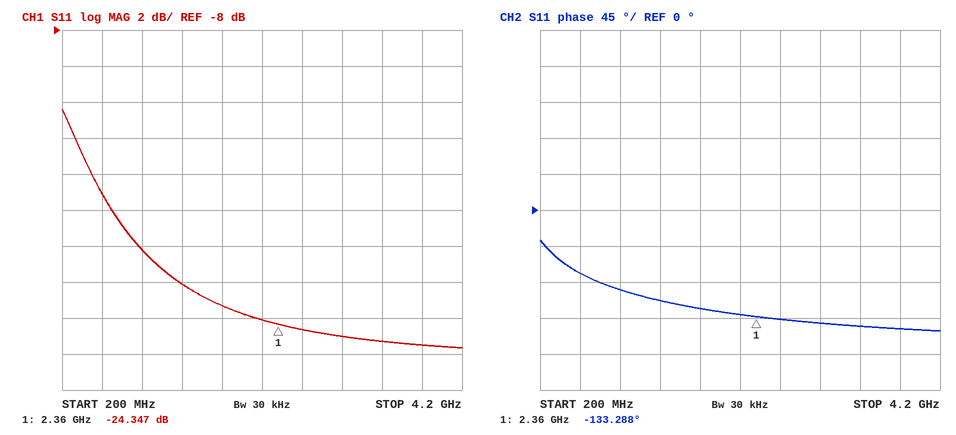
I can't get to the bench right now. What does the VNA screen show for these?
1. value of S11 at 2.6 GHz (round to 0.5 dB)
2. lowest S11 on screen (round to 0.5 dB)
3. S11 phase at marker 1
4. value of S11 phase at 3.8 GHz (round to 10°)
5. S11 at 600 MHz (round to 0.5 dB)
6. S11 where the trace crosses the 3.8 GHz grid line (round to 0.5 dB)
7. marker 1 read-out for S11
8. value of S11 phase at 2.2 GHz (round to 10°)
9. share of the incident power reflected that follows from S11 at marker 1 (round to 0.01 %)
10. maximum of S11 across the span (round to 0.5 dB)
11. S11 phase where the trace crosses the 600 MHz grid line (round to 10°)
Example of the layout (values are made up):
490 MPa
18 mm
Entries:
-24.5 dB
-25.5 dB
-133.288°
-150°
-17.0 dB
-25.5 dB
-24.347 dB
-130°
0.37 %
-12.5 dB
-80°
